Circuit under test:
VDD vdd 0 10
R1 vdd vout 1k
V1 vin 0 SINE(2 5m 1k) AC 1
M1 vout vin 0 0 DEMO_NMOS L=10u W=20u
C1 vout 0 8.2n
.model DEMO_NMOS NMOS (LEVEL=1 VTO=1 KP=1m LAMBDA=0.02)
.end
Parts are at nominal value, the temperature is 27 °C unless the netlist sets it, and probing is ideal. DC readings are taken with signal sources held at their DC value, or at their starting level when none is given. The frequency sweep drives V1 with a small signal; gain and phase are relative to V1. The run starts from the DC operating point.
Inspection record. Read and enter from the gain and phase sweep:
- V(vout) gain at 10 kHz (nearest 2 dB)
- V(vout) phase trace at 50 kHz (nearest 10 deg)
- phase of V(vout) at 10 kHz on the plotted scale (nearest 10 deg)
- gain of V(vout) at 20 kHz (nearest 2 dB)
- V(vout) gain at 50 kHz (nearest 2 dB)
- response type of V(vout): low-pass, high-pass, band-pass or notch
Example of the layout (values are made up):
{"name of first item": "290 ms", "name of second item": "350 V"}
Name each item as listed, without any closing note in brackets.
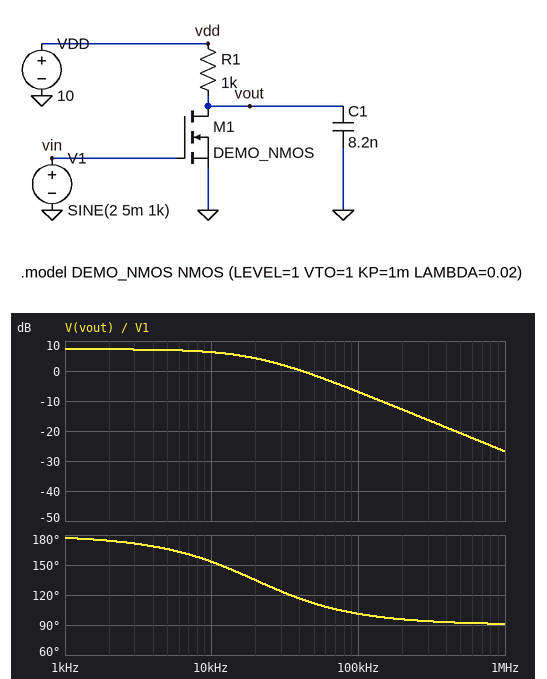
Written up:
{"V(vout) gain at 10 kHz": "6 dB", "V(vout) phase trace at 50 kHz": "110 deg", "phase of V(vout) at 10 kHz on the plotted scale": "150 deg", "gain of V(vout) at 20 kHz": "4 dB", "V(vout) gain at 50 kHz": "-2 dB", "response type of V(vout): low-pass, high-pass, band-pass or notch": "low-pass"}
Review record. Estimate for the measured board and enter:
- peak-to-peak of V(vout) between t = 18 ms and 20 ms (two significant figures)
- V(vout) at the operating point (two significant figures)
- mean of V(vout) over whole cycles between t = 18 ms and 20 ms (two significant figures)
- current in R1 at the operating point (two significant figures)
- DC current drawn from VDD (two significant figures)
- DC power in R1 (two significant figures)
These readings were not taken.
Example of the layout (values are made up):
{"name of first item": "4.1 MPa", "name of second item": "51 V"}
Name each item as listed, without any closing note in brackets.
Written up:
{"peak-to-peak of V(vout) between t = 18 ms and 20 ms": "23 mV", "V(vout) at the operating point": "8.8 V", "mean of V(vout) over whole cycles between t = 18 ms and 20 ms": "8.8 V", "current in R1 at the operating point": "1.2 mA", "DC current drawn from VDD": "1.2 mA", "DC power in R1": "1.4 mW"}
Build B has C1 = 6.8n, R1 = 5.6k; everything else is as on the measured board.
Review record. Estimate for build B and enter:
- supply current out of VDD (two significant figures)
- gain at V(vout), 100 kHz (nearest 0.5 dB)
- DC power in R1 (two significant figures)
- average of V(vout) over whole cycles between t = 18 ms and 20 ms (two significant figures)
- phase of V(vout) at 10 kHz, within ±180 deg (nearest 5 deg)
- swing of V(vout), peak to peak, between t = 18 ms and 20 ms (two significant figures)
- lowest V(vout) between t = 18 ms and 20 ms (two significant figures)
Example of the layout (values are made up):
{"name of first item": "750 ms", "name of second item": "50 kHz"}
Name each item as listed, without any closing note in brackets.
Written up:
{"supply current out of VDD": "1.1 mA", "gain at V(vout), 100 kHz": "-6.0 dB", "DC power in R1": "6.5 mW", "average of V(vout) over whole cycles between t = 18 ms and 20 ms": "4.0 V", "phase of V(vout) at 10 kHz, within ±180 deg": "115 deg", "swing of V(vout), peak to peak, between t = 18 ms and 20 ms": "110 mV", "lowest V(vout) between t = 18 ms and 20 ms": "3.9 V"}
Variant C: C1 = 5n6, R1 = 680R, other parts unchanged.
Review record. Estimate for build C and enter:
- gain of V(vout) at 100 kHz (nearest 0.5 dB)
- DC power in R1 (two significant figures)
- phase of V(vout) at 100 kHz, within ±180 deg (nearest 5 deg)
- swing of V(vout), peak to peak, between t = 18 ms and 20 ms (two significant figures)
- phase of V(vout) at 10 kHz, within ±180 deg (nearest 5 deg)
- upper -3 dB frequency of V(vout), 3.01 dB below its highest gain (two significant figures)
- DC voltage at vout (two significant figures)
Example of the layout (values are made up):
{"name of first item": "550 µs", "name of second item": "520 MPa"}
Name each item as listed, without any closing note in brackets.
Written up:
{"gain of V(vout) at 100 kHz": "-4.0 dB", "DC power in R1": "950 µW", "phase of V(vout) at 100 kHz, within ±180 deg": "115 deg", "swing of V(vout), peak to peak, between t = 18 ms and 20 ms": "16 mV", "phase of V(vout) at 10 kHz, within ±180 deg": "165 deg", "upper -3 dB frequency of V(vout), 3.01 dB below its highest gain": "42 kHz", "DC voltage at vout": "9.2 V"}
